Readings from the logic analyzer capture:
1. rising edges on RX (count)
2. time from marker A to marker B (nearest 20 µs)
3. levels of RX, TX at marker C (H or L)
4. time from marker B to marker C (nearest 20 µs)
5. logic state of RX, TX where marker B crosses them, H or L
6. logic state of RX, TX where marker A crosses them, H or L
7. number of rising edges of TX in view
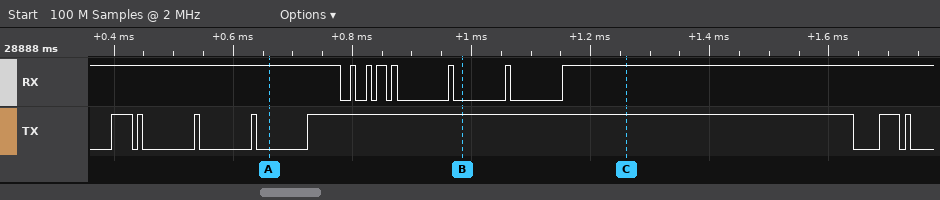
7
320 µs
RX=H, TX=H
280 µs
RX=L, TX=H
RX=H, TX=L
7
